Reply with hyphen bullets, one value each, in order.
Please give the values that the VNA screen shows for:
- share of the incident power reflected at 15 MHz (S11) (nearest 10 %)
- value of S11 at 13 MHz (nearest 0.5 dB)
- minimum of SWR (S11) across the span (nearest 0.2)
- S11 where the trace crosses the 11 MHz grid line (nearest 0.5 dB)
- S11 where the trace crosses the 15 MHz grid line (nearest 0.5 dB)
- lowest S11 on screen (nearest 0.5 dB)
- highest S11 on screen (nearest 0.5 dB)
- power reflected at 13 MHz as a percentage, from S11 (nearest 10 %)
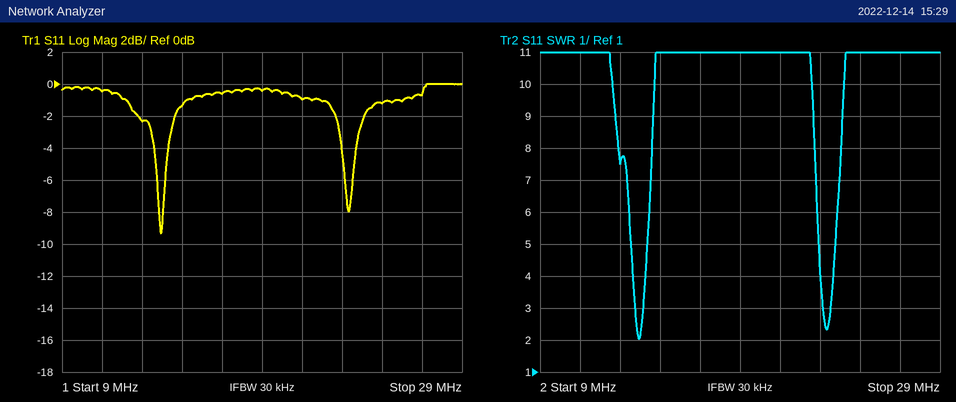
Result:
- 70 %
- -2.5 dB
- 2.0
- -0.5 dB
- -1.5 dB
- -9.5 dB
- 0.0 dB
- 60 %
